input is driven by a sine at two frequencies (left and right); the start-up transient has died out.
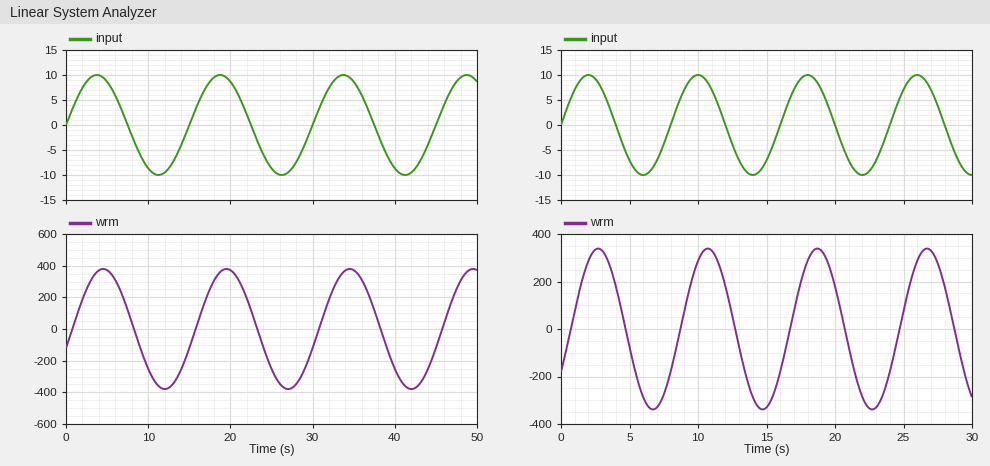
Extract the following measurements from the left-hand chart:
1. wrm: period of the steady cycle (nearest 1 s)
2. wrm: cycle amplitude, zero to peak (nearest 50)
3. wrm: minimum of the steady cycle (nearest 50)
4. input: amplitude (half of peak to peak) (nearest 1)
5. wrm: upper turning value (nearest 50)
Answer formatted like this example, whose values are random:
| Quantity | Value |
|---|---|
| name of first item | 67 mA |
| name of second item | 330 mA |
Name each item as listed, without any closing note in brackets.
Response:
| Quantity | Value |
|---|---|
| wrm: period of the steady cycle | 15 s |
| wrm: cycle amplitude, zero to peak | 400 |
| wrm: minimum of the steady cycle | -400 |
| input: amplitude (half of peak to peak) | 10 |
| wrm: upper turning value | 400 |
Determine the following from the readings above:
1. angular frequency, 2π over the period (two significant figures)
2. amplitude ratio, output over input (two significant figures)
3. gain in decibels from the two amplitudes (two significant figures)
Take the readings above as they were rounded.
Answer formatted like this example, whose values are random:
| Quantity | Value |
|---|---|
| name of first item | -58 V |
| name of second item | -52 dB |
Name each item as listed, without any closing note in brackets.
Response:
| Quantity | Value |
|---|---|
| angular frequency, 2π over the period | 0.42 rad/s |
| amplitude ratio, output over input | 40 |
| gain in decibels from the two amplitudes | 32 dB |
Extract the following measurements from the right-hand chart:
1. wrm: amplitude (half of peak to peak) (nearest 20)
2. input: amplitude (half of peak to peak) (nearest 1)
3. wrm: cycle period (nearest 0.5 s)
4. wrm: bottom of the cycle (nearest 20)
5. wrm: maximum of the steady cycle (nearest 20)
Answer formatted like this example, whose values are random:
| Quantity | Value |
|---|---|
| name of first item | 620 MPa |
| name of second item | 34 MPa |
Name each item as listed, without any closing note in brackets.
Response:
| Quantity | Value |
|---|---|
| wrm: amplitude (half of peak to peak) | 340 |
| input: amplitude (half of peak to peak) | 10 |
| wrm: cycle period | 8.0 s |
| wrm: bottom of the cycle | -340 |
| wrm: maximum of the steady cycle | 340 |
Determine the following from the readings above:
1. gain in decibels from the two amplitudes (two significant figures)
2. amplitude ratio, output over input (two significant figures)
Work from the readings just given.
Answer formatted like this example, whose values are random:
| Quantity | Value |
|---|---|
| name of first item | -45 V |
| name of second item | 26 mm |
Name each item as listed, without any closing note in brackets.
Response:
| Quantity | Value |
|---|---|
| gain in decibels from the two amplitudes | 31 dB |
| amplitude ratio, output over input | 34 |
